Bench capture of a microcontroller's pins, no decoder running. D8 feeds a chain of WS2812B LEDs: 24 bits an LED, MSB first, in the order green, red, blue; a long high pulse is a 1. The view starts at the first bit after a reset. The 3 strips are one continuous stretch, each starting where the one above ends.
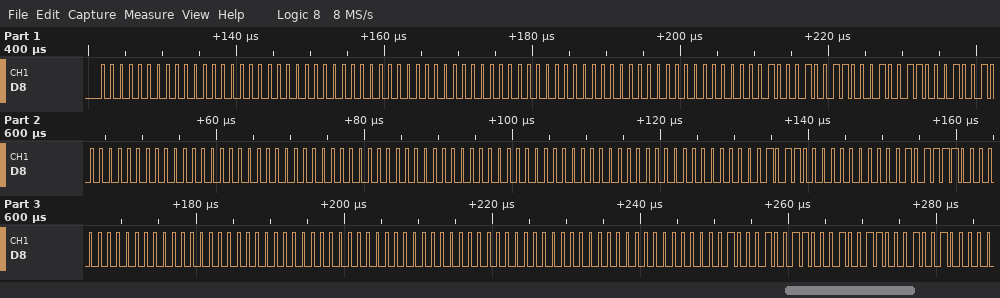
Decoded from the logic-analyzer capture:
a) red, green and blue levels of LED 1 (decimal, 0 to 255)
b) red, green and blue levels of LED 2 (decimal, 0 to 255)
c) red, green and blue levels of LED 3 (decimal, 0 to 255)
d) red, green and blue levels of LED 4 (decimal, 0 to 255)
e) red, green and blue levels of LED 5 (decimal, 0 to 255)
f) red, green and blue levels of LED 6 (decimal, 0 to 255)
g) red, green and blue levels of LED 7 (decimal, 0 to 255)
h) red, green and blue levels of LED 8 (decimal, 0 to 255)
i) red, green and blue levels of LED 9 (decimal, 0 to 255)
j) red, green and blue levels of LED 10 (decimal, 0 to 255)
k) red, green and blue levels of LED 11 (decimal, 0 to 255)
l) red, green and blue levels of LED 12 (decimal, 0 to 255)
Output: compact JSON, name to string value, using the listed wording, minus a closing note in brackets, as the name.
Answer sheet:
{"red, green and blue levels of LED 1": "0, 0, 0", "red, green and blue levels of LED 2": "0, 0, 0", "red, green and blue levels of LED 3": "0, 0, 0", "red, green and blue levels of LED 4": "137, 137, 137", "red, green and blue levels of LED 5": "0, 0, 0", "red, green and blue levels of LED 6": "0, 0, 0", "red, green and blue levels of LED 7": "0, 0, 0", "red, green and blue levels of LED 8": "0, 44, 94", "red, green and blue levels of LED 9": "0, 0, 0", "red, green and blue levels of LED 10": "0, 0, 0", "red, green and blue levels of LED 11": "0, 0, 0", "red, green and blue levels of LED 12": "137, 137, 137"}
